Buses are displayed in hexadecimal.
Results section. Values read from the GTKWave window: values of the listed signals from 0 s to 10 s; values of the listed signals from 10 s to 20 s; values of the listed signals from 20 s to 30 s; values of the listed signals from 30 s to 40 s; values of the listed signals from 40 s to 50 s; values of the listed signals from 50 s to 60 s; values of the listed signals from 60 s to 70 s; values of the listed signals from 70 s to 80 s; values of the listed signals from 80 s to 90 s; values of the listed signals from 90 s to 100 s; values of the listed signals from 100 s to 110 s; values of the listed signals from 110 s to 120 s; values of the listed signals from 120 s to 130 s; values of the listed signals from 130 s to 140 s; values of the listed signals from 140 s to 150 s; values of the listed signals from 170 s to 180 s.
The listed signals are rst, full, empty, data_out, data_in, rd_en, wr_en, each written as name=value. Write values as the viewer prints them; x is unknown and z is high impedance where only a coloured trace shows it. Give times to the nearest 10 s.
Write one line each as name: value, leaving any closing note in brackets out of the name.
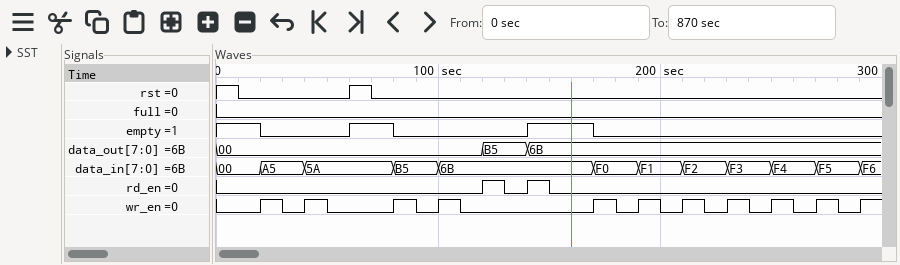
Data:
values of the listed signals from 0 s to 10 s: rst=1, full=0, empty=1, data_out=00, data_in=00, rd_en=0, wr_en=0
values of the listed signals from 10 s to 20 s: rst=0, full=0, empty=1, data_out=00, data_in=00, rd_en=0, wr_en=0
values of the listed signals from 20 s to 30 s: rst=0, full=0, empty=0, data_out=00, data_in=A5, rd_en=0, wr_en=1
values of the listed signals from 30 s to 40 s: rst=0, full=0, empty=0, data_out=00, data_in=A5, rd_en=0, wr_en=0
values of the listed signals from 40 s to 50 s: rst=0, full=0, empty=0, data_out=00, data_in=5A, rd_en=0, wr_en=1
values of the listed signals from 50 s to 60 s: rst=0, full=0, empty=0, data_out=00, data_in=5A, rd_en=0, wr_en=0
values of the listed signals from 60 s to 70 s: rst=1, full=0, empty=1, data_out=00, data_in=5A, rd_en=0, wr_en=0
values of the listed signals from 70 s to 80 s: rst=0, full=0, empty=1, data_out=00, data_in=5A, rd_en=0, wr_en=0
values of the listed signals from 80 s to 90 s: rst=0, full=0, empty=0, data_out=00, data_in=B5, rd_en=0, wr_en=1
values of the listed signals from 90 s to 100 s: rst=0, full=0, empty=0, data_out=00, data_in=B5, rd_en=0, wr_en=0
values of the listed signals from 100 s to 110 s: rst=0, full=0, empty=0, data_out=00, data_in=6B, rd_en=0, wr_en=1
values of the listed signals from 110 s to 120 s: rst=0, full=0, empty=0, data_out=00, data_in=6B, rd_en=0, wr_en=0
values of the listed signals from 120 s to 130 s: rst=0, full=0, empty=0, data_out=B5, data_in=6B, rd_en=1, wr_en=0
values of the listed signals from 130 s to 140 s: rst=0, full=0, empty=0, data_out=B5, data_in=6B, rd_en=0, wr_en=0
values of the listed signals from 140 s to 150 s: rst=0, full=0, empty=1, data_out=6B, data_in=6B, rd_en=1, wr_en=0
values of the listed signals from 170 s to 180 s: rst=0, full=0, empty=0, data_out=6B, data_in=F0, rd_en=0, wr_en=1
